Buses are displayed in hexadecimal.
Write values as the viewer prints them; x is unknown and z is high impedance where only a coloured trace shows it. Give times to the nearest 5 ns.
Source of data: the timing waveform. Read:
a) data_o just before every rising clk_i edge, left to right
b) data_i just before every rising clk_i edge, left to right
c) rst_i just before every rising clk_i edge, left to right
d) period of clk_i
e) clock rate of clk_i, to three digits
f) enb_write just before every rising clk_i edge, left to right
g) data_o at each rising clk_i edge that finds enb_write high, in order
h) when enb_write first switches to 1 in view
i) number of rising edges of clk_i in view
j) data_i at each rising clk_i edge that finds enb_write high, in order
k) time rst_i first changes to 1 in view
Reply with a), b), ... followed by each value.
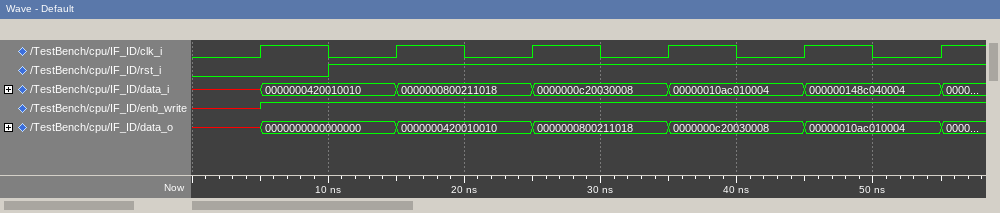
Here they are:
a) x, 0000000000000000, 0000000420010010, 0000000800211018, 0000000c20030008, 00000010ac010004
b) x, 0000000420010010, 0000000800211018, 0000000c20030008, 00000010ac010004, 000000148c040004
c) 0 1 1 1 1 1
d) 10 ns
e) 100 MHz
f) x 1 1 1 1 1
g) 0000000000000000, 0000000420010010, 0000000800211018, 0000000c20030008, 00000010ac010004
h) 5 ns
i) 6
j) 0000000420010010, 0000000800211018, 0000000c20030008, 00000010ac010004, 000000148c040004
k) 10 ns
